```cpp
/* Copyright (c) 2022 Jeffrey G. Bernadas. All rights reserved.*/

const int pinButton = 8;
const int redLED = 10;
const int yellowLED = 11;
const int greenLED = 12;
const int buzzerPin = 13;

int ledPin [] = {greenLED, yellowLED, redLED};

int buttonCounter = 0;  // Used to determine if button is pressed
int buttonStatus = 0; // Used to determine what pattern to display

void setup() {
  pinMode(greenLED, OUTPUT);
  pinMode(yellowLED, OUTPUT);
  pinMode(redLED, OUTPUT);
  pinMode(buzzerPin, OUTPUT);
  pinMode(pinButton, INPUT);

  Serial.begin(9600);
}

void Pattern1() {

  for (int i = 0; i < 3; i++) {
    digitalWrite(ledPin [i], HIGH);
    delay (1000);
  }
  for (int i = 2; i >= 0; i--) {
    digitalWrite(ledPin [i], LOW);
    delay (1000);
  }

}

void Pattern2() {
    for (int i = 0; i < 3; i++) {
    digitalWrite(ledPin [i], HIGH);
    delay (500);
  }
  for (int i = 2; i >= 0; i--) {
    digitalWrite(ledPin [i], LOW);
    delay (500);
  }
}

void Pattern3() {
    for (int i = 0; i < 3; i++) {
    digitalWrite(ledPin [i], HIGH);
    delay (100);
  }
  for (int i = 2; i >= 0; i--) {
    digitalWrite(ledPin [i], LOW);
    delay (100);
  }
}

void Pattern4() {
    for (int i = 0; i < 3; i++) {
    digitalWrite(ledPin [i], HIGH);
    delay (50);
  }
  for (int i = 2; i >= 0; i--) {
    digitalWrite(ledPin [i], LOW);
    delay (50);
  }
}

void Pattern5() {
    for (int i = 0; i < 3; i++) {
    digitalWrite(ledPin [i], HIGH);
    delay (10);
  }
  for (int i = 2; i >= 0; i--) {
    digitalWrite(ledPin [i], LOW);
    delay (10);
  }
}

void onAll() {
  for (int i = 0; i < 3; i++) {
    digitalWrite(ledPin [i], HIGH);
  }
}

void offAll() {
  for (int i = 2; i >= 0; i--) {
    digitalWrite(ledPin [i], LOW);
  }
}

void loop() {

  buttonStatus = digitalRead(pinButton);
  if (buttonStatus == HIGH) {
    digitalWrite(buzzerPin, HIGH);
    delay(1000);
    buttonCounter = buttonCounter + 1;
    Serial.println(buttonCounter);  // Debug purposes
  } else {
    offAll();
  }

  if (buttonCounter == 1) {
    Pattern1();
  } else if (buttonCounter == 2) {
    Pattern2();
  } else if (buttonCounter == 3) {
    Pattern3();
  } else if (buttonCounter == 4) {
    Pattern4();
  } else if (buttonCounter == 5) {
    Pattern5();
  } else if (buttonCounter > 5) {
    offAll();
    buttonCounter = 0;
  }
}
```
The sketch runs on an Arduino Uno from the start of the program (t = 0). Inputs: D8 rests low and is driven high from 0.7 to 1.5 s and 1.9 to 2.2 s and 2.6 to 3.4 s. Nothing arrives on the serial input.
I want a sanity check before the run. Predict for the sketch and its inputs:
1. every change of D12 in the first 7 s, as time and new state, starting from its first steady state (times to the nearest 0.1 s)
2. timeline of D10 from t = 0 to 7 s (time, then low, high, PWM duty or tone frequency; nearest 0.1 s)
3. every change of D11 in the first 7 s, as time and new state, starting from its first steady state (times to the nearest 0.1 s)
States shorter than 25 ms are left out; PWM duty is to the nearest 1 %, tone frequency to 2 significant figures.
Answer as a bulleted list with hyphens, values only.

- 0 s low; 1.7 s high; 6.7 s low
- 0 s low; 3.7 s high; 4.7 s low
- 0 s low; 2.7 s high; 5.7 s low
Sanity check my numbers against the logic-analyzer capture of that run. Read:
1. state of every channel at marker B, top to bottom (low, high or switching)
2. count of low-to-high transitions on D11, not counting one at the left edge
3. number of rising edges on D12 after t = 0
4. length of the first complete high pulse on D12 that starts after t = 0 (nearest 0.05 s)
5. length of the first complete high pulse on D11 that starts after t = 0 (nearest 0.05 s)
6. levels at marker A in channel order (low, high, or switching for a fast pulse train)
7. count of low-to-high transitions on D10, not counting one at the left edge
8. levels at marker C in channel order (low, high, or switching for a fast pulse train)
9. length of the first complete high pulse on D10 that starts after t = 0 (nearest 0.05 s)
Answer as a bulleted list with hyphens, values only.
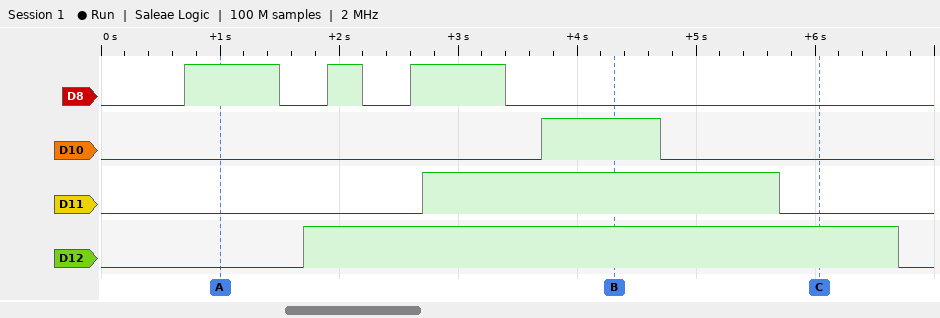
- D8 low, D10 high, D11 high, D12 high
- 1
- 1
- 5.00 s
- 3.00 s
- D8 high, D10 low, D11 low, D12 low
- 1
- D8 low, D10 low, D11 low, D12 high
- 1.00 s
